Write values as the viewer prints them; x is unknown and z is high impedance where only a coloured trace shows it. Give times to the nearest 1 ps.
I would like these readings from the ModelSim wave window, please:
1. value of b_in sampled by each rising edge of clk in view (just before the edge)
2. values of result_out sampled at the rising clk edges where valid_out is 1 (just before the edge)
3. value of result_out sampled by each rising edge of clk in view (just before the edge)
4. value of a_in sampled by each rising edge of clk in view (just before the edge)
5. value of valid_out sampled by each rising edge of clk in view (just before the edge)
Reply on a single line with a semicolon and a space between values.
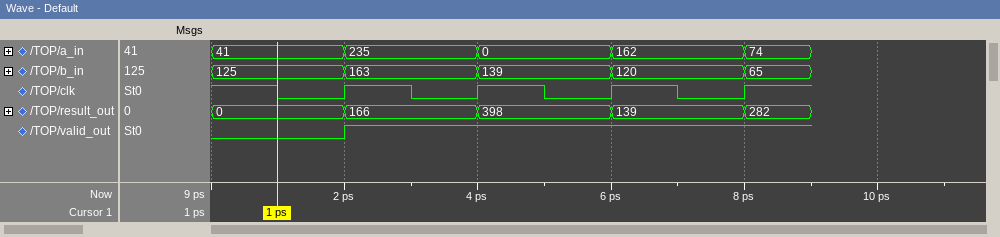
125, 163, 139, 120; 166, 398, 139; 0, 166, 398, 139; 41, 235, 0, 162; 0 1 1 1
